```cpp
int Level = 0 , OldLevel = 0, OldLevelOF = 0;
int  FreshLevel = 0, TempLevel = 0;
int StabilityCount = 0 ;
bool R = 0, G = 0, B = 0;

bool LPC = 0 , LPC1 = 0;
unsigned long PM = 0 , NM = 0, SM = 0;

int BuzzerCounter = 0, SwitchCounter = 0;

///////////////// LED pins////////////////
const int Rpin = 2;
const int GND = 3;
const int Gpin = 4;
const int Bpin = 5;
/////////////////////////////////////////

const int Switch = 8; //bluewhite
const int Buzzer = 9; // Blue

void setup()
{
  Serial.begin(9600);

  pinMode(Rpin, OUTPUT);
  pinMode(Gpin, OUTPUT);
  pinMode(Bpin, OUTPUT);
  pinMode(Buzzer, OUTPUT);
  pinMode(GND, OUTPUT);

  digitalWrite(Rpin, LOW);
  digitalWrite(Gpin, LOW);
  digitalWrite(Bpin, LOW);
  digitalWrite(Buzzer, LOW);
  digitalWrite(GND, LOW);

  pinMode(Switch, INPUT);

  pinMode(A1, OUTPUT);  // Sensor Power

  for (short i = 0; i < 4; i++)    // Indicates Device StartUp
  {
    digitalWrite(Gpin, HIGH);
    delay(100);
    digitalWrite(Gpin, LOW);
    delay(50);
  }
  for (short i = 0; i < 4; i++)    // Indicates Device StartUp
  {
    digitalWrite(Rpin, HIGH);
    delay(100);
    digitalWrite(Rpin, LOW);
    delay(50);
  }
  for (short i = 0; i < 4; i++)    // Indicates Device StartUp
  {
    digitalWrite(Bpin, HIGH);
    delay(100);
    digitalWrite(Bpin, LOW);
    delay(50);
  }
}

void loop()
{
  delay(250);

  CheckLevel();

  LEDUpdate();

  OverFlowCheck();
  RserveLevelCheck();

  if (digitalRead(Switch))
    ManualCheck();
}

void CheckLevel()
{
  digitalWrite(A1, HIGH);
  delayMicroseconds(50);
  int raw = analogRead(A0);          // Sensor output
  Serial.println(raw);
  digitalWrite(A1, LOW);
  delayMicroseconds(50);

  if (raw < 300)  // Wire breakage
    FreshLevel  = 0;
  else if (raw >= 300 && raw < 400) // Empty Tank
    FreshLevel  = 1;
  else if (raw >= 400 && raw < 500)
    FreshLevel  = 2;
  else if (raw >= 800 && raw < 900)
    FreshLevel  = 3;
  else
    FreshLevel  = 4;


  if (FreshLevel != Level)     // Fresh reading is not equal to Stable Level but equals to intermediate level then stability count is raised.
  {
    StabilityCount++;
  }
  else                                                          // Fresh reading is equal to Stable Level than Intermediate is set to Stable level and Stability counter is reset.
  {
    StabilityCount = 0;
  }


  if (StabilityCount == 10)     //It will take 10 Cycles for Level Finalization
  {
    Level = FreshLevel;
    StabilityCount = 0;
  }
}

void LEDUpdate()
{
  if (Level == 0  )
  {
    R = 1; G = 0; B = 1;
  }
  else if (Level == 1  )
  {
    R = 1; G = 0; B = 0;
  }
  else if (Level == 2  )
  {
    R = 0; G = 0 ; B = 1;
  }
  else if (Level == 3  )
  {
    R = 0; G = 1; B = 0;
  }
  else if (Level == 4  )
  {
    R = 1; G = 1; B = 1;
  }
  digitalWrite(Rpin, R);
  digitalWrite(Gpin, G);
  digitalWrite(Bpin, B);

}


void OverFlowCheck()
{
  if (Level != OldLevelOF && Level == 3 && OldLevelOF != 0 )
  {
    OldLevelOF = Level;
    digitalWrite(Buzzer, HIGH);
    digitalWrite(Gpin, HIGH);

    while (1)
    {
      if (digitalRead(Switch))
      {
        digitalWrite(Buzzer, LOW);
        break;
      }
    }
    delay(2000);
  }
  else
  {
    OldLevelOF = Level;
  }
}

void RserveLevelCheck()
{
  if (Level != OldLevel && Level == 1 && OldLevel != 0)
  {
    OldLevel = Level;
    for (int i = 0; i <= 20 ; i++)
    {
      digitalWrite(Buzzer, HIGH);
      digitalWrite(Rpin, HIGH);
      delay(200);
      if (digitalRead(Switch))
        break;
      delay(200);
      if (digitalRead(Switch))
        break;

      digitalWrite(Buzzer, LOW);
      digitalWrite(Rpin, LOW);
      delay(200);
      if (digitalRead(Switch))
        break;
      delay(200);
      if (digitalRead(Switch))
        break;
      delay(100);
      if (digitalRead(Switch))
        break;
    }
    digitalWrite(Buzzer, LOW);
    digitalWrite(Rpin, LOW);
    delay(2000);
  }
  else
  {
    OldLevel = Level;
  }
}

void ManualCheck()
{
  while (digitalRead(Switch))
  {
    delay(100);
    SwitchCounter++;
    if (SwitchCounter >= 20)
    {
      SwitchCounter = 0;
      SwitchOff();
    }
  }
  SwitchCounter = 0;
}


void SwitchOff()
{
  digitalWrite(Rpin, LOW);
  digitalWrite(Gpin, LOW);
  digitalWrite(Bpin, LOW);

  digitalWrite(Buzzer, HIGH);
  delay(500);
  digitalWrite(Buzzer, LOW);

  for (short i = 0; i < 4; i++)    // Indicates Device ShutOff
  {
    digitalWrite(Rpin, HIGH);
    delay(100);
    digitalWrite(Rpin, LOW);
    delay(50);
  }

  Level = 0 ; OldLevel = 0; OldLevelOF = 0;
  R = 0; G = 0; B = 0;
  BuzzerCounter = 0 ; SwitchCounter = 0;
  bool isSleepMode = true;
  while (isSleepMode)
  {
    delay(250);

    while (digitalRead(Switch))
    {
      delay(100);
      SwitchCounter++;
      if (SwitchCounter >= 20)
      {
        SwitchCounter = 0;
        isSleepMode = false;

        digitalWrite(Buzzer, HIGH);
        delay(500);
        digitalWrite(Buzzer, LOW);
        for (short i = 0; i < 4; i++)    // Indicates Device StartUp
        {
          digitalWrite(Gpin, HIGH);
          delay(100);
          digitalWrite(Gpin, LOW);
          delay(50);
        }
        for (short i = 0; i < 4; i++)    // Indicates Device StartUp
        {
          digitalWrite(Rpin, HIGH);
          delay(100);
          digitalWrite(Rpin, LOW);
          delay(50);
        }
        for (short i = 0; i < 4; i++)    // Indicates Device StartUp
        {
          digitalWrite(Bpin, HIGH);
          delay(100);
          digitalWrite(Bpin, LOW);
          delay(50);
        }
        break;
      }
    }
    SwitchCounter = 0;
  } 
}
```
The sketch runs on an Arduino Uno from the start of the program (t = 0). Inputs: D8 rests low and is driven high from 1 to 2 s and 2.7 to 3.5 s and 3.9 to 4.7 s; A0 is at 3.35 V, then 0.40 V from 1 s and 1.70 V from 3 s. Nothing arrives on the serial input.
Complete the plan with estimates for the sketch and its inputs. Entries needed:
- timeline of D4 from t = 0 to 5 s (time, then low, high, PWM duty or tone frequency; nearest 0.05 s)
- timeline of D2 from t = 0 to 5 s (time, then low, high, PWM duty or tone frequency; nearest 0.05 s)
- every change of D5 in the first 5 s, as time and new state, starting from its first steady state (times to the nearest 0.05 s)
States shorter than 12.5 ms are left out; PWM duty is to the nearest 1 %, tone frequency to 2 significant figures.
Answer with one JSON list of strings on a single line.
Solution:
["0 s high; 0.1 s low; 0.15 s high; 0.25 s low; 0.3 s high; 0.4 s low; 0.45 s high; 0.55 s low", "0 s low; 0.6 s high; 0.7 s low; 0.75 s high; 0.85 s low; 0.9 s high; 1 s low; 1.05 s high; 1.15 s low; 2.05 s high", "0 s low; 1.2 s high; 1.3 s low; 1.35 s high; 1.45 s low; 1.5 s high; 1.6 s low; 1.65 s high; 1.75 s low; 2.05 s high"]
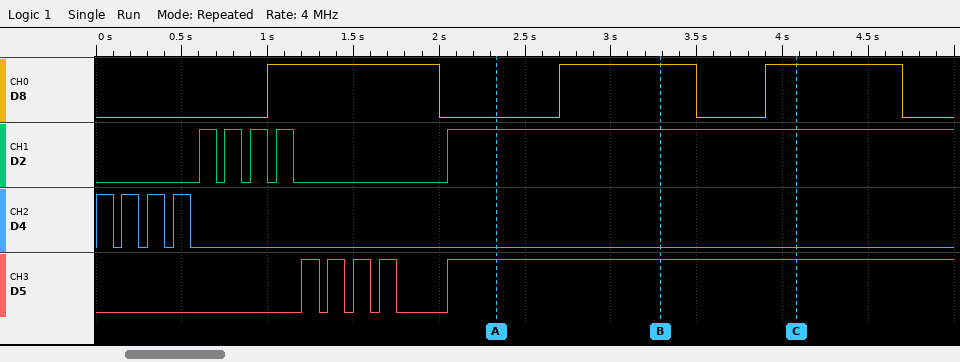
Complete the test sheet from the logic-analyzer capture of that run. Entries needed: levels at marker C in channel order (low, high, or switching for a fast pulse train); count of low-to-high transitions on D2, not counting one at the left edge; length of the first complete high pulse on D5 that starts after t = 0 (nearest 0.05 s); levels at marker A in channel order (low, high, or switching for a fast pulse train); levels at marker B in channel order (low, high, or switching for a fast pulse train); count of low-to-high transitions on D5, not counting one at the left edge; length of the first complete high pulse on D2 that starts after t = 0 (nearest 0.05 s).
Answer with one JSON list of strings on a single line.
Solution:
["D8 high, D2 high, D4 low, D5 high", "5", "0.10 s", "D8 low, D2 high, D4 low, D5 high", "D8 high, D2 high, D4 low, D5 high", "5", "0.10 s"]
